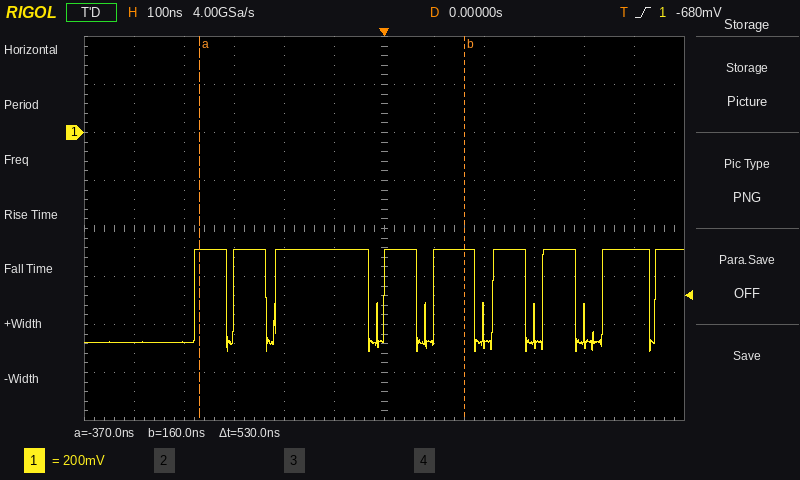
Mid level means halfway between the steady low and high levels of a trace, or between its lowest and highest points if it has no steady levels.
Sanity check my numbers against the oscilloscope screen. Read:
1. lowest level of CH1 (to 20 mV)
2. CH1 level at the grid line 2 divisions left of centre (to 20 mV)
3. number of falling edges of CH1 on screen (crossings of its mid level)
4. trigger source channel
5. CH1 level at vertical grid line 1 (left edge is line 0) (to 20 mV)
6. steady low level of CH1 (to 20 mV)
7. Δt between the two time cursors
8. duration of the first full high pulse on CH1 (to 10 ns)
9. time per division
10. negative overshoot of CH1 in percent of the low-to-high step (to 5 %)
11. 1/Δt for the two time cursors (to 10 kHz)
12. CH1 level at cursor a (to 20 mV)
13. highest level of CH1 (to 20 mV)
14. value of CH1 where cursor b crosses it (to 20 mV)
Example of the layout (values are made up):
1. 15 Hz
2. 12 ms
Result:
1. -920 mV
2. -480 mV
3. 8
4. CH1
5. -880 mV
6. -880 mV
7. 530 ns
8. 60 ns
9. 100 ns
10. 10 %
11. 1.89 MHz
12. -480 mV
13. -480 mV
14. -480 mV
